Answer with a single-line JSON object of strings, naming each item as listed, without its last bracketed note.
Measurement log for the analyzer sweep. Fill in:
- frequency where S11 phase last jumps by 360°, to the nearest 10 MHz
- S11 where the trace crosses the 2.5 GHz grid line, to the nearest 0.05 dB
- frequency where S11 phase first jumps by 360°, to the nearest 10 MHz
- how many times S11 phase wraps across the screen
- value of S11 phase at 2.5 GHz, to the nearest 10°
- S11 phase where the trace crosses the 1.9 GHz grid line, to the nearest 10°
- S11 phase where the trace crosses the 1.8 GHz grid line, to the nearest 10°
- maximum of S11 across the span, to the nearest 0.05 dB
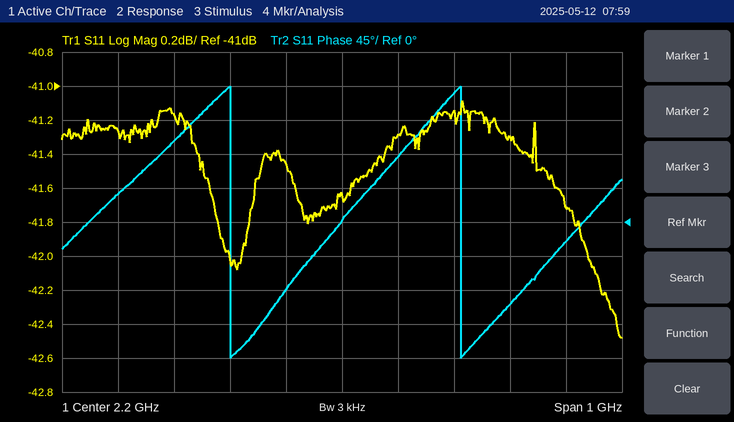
{"frequency where S11 phase last jumps by 360°, to the nearest 10 MHz": "2.41 GHz", "S11 where the trace crosses the 2.5 GHz grid line, to the nearest 0.05 dB": "-41.30 dB", "frequency where S11 phase first jumps by 360°, to the nearest 10 MHz": "2.00 GHz", "how many times S11 phase wraps across the screen": "2", "value of S11 phase at 2.5 GHz, to the nearest 10°": "-110°", "S11 phase where the trace crosses the 1.9 GHz grid line, to the nearest 10°": "110°", "S11 phase where the trace crosses the 1.8 GHz grid line, to the nearest 10°": "40°", "maximum of S11 across the span, to the nearest 0.05 dB": "-41.10 dB"}
